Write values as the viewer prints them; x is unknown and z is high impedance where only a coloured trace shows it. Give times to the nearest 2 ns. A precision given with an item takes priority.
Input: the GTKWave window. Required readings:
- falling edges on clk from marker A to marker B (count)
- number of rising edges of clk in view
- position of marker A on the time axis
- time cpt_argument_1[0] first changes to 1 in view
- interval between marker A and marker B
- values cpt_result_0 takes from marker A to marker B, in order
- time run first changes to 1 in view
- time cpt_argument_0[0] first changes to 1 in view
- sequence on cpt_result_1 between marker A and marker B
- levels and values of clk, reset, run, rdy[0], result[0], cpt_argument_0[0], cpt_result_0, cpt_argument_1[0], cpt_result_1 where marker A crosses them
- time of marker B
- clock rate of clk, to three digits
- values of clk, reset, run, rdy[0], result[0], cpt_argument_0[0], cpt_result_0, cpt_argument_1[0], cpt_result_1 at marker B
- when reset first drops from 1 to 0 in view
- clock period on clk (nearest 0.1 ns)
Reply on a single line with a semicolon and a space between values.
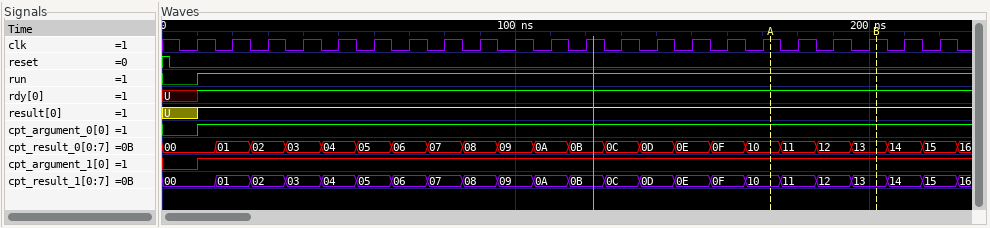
3; 22; 172 ns; 10 ns; 30 ns; 10, 11, 12, 13; 10 ns; 10 ns; 10, 11, 12, 13; clk=1, reset=0, run=1, rdy[0]=1, result[0]=1, cpt_argument_0[0]=1, cpt_result_0=10, cpt_argument_1[0]=1, cpt_result_1=10; 202 ns; 100 MHz; clk=1, reset=0, run=1, rdy[0]=1, result[0]=1, cpt_argument_0[0]=1, cpt_result_0=13, cpt_argument_1[0]=1, cpt_result_1=13; 2 ns; 10 ns
